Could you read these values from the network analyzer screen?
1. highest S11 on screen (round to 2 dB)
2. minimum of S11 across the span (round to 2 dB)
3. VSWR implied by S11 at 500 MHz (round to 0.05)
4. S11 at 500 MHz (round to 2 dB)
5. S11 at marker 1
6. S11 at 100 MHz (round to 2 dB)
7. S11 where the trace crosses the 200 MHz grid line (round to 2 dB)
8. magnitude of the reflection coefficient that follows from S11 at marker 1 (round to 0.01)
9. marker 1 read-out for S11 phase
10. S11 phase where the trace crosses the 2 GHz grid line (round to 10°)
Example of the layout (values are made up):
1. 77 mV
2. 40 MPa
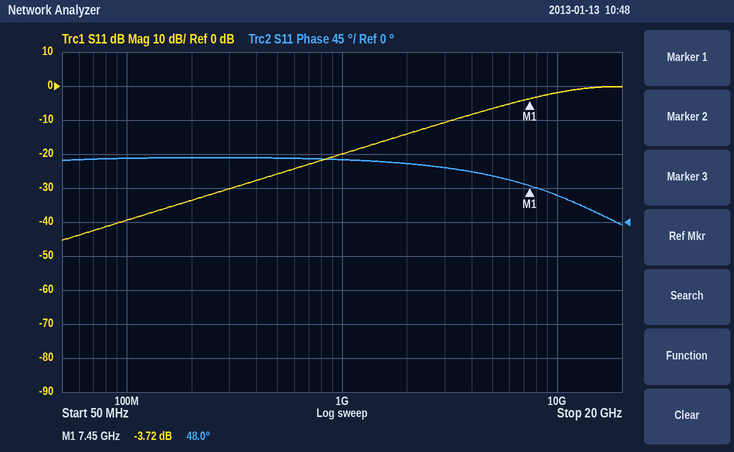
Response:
1. 0 dB
2. -46 dB
3. 1.10
4. -26 dB
5. -3.72 dB
6. -40 dB
7. -34 dB
8. 0.65
9. 48.0°
10. 80°
